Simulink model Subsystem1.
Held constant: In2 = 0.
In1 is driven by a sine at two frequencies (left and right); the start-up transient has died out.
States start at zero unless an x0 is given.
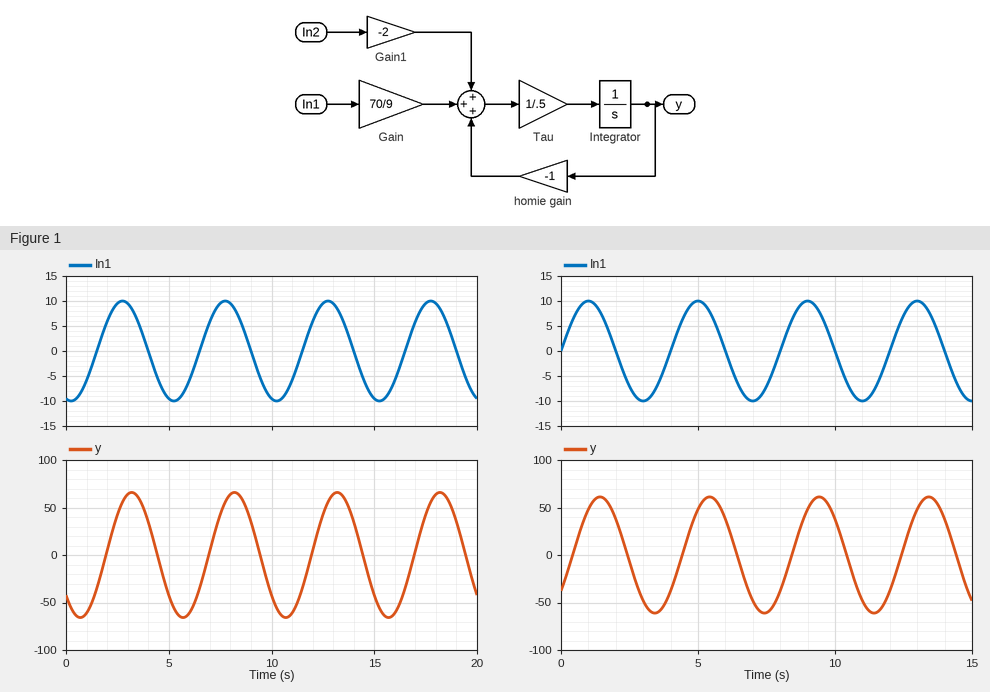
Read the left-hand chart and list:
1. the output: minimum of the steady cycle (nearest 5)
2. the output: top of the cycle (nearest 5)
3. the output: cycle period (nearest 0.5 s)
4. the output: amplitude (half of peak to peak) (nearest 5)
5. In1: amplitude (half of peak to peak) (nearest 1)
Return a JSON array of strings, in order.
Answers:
["-65", "65", "5.0 s", "65", "10"]
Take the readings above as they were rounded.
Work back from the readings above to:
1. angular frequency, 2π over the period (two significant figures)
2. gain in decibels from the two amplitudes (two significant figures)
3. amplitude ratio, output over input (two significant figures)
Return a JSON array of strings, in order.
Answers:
["1.3 rad/s", "16 dB", "6.5"]
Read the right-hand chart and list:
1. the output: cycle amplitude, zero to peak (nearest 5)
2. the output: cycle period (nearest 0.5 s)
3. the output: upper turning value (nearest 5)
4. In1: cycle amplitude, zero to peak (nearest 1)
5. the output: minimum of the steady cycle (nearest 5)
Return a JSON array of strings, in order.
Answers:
["60", "4.0 s", "60", "10", "-60"]
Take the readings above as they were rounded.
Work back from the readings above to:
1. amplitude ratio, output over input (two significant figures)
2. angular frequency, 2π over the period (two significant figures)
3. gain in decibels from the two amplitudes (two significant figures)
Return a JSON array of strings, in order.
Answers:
["6.0", "1.6 rad/s", "16 dB"]
